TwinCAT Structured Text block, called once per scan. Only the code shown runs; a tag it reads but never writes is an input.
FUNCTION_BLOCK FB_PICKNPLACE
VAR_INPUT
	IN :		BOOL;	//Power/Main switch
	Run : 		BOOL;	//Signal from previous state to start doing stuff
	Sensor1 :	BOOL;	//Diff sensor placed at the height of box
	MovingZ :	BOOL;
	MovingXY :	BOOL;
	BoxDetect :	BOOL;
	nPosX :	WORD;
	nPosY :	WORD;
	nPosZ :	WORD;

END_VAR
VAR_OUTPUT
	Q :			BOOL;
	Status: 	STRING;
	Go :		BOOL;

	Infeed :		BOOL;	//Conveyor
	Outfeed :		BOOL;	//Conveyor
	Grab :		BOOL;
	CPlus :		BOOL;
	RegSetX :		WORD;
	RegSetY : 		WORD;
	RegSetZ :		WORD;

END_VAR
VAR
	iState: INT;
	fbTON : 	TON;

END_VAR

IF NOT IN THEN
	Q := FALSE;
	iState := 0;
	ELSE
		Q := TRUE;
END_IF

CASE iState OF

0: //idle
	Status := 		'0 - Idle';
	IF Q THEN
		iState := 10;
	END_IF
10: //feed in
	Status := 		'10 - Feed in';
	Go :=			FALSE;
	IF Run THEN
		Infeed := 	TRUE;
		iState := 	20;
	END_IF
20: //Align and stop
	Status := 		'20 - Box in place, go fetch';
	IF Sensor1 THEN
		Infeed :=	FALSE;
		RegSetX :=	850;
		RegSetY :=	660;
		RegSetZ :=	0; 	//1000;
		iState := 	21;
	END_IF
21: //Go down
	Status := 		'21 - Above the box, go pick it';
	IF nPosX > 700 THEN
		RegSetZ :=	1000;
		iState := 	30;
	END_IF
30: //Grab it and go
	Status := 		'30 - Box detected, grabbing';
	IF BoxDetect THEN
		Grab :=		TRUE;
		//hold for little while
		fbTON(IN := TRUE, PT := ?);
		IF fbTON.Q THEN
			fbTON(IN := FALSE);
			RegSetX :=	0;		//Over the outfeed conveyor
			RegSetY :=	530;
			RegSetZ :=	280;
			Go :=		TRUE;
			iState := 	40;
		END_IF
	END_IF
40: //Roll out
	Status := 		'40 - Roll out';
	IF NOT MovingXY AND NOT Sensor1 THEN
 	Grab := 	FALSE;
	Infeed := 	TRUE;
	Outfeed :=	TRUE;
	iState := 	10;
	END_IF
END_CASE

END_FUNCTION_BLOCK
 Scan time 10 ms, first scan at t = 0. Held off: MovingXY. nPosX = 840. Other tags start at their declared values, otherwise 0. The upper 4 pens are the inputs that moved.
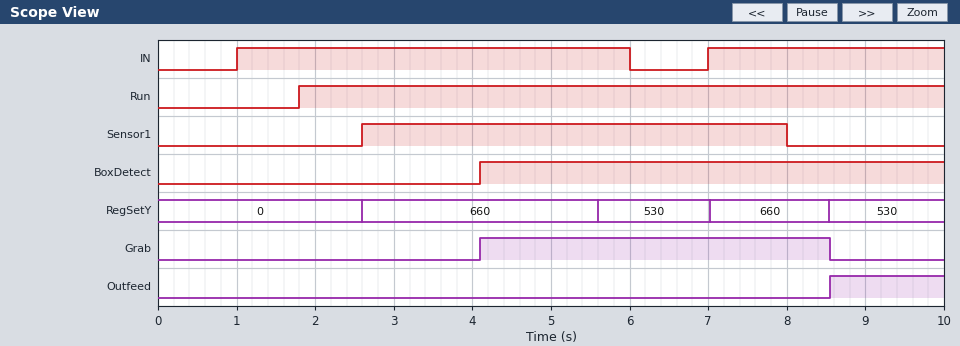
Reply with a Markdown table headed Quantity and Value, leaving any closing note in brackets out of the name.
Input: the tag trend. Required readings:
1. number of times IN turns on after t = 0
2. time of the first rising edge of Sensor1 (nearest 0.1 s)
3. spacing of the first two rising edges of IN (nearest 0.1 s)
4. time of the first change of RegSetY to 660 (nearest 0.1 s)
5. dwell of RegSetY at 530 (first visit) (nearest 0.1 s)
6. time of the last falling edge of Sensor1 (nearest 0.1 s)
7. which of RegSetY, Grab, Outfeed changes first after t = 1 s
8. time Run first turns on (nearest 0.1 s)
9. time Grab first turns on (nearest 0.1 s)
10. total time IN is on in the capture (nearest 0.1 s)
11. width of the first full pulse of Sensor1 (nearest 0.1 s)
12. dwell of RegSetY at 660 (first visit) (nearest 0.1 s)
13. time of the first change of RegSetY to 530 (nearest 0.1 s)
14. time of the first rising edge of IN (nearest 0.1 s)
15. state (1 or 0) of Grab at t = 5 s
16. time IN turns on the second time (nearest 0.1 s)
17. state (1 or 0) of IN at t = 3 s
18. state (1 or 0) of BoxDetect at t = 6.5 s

| Quantity | Value |
|---|---|
| number of times IN turns on after t = 0 | 2 |
| time of the first rising edge of Sensor1 | 2.6 s |
| spacing of the first two rising edges of IN | 6.0 s |
| time of the first change of RegSetY to 660 | 2.6 s |
| dwell of RegSetY at 530 (first visit) | 1.4 s |
| time of the last falling edge of Sensor1 | 8.0 s |
| which of RegSetY, Grab, Outfeed changes first after t = 1 s | RegSetY |
| time Run first turns on | 1.8 s |
| time Grab first turns on | 4.1 s |
| total time IN is on in the capture | 8.0 s |
| width of the first full pulse of Sensor1 | 5.4 s |
| dwell of RegSetY at 660 (first visit) | 3.0 s |
| time of the first change of RegSetY to 530 | 5.6 s |
| time of the first rising edge of IN | 1.0 s |
| state (1 or 0) of Grab at t = 5 s | 1 |
| time IN turns on the second time | 7.0 s |
| state (1 or 0) of IN at t = 3 s | 1 |
| state (1 or 0) of BoxDetect at t = 6.5 s | 1 |
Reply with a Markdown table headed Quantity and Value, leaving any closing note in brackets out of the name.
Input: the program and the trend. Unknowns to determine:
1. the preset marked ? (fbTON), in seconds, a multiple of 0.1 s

| Quantity | Value |
|---|---|
| the preset marked ? (fbTON), in seconds, a multiple of 0.1 s | 1.5 s |
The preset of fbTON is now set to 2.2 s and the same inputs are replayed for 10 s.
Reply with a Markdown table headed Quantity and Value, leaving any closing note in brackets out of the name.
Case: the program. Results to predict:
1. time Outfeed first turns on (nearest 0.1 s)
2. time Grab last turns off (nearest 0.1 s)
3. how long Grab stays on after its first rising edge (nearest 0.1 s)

| Quantity | Value |
|---|---|
| time Outfeed first turns on | 8.0 s |
| time Grab last turns off | 8.0 s |
| how long Grab stays on after its first rising edge | 3.9 s |
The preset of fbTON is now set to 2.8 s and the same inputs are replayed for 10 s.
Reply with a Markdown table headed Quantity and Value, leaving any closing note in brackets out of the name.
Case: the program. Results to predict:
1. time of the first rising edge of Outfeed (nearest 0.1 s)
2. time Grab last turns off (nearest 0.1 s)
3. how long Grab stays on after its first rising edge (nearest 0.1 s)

| Quantity | Value |
|---|---|
| time of the first rising edge of Outfeed | 8.0 s |
| time Grab last turns off | 8.0 s |
| how long Grab stays on after its first rising edge | 3.9 s |
